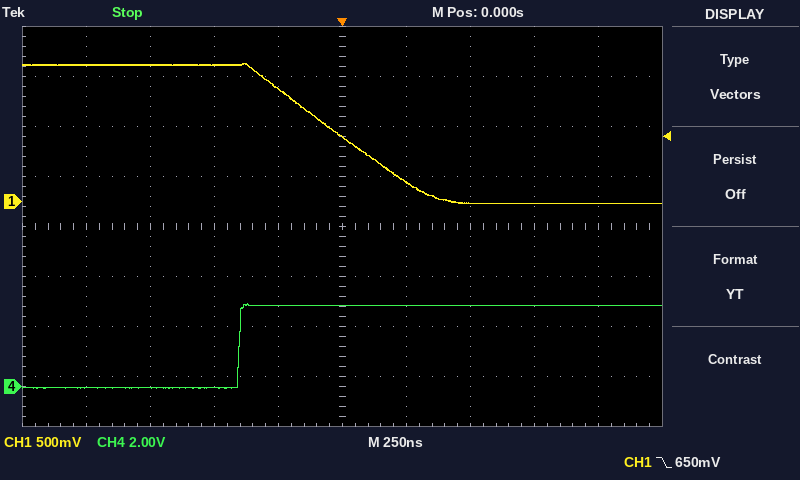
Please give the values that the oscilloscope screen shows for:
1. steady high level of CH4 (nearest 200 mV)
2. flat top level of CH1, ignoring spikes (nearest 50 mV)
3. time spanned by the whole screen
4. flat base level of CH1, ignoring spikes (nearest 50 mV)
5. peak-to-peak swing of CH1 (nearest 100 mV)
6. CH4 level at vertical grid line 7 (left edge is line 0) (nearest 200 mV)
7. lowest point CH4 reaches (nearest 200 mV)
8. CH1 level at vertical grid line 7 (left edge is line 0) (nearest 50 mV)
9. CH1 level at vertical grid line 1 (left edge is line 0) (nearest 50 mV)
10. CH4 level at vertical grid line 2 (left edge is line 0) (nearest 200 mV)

3.2 V
1.35 V
2.5 µs
0 mV
1.40 V
3.2 V
0.0 V
0 mV
1.35 V
0.0 V
